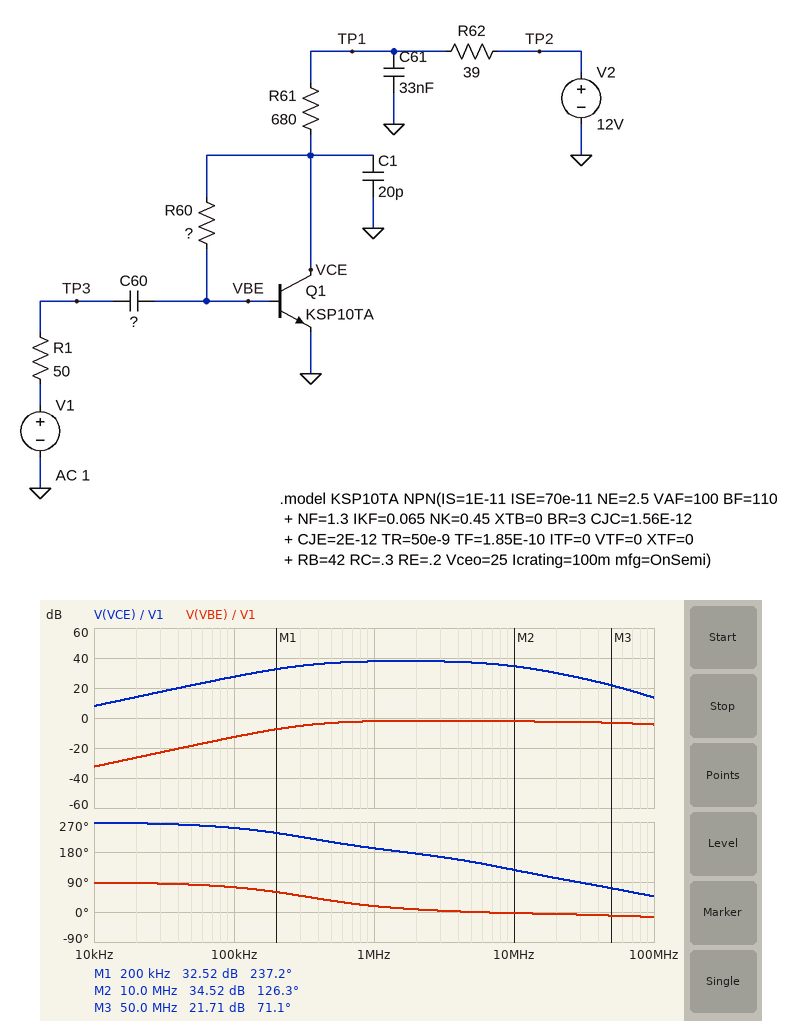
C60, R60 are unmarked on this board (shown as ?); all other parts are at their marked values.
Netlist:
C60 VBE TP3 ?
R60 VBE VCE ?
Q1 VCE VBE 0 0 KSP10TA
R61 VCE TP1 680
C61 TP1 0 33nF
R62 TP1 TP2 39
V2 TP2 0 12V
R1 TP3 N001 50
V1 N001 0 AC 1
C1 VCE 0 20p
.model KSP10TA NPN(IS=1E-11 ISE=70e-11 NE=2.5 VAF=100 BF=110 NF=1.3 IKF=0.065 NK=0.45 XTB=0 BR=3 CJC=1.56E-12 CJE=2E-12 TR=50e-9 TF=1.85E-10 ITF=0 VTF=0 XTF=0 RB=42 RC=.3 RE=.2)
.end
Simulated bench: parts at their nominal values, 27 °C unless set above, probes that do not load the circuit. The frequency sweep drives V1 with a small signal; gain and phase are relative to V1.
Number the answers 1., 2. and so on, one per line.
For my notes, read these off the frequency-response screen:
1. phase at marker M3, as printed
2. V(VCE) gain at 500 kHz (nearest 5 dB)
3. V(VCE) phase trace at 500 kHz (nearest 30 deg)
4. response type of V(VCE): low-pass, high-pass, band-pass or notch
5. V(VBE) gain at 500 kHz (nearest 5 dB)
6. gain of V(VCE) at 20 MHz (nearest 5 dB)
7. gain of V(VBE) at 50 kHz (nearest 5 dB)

1. 71.1 deg
2. 35 dB
3. 210 deg
4. band-pass
5. -5 dB
6. 30 dB
7. -20 dB
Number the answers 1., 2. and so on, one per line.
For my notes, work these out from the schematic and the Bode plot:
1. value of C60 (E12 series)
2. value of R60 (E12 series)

1. 1.2 nF
2. 82 kΩ
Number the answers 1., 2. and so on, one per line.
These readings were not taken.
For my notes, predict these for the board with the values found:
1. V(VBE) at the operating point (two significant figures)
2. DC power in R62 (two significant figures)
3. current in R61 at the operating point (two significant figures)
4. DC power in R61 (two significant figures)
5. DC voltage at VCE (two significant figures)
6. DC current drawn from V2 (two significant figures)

1. 690 mV
2. 1.5 mW
3. 6.3 mA
4. 27 mW
5. 7.5 V
6. 6.3 mA
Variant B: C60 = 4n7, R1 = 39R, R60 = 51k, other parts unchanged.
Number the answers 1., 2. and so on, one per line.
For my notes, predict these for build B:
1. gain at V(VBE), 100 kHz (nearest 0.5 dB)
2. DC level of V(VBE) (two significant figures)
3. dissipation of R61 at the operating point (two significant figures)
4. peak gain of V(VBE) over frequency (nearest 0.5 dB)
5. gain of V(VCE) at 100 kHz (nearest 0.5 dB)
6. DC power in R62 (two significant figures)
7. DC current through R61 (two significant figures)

1. -6.0 dB
2. 700 mV
3. 45 mW
4. -1.5 dB
5. 36.0 dB
6. 2.6 mW
7. 8.1 mA
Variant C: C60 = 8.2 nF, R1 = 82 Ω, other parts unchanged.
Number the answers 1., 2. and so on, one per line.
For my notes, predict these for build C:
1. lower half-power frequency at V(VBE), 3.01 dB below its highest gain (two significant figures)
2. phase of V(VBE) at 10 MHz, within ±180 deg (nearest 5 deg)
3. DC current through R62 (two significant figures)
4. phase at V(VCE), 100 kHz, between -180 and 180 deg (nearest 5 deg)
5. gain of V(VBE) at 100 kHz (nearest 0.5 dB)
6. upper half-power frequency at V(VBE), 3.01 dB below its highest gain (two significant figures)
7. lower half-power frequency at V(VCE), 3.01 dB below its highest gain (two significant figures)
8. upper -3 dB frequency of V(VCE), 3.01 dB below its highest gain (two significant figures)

1. 48 kHz
2. -10 deg
3. 6.3 mA
4. -155 deg
5. -3.0 dB
6. 58 MHz
7. 44 kHz
8. 7.8 MHz
